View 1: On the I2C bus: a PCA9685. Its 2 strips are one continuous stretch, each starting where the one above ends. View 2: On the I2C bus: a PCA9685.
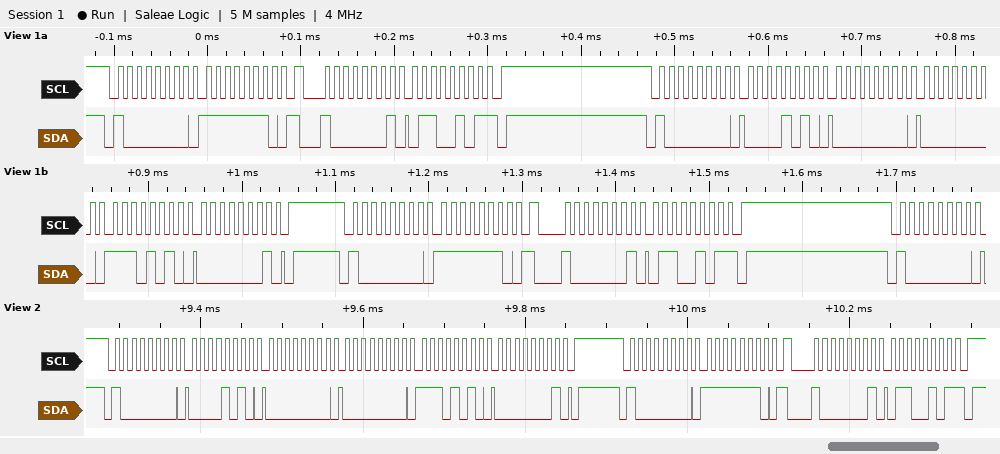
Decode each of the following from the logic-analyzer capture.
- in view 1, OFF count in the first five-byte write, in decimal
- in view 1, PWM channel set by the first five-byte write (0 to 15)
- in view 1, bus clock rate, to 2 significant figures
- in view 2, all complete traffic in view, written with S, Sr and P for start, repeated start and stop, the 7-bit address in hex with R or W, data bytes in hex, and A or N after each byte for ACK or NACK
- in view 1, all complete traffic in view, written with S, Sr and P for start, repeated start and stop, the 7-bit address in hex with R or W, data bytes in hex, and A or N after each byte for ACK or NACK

490
1
100 kHz
S 40W A 0A A 00 A 00 A EA A 01 A P S 40W A FE A Sr 40R A 65 N P
S 40W A FE A Sr 40R A 65 N P S 40W A 0A A 00 A 00 A EA A 01 A P S 40W A FE A Sr 40R A 65 N P S 40W A
